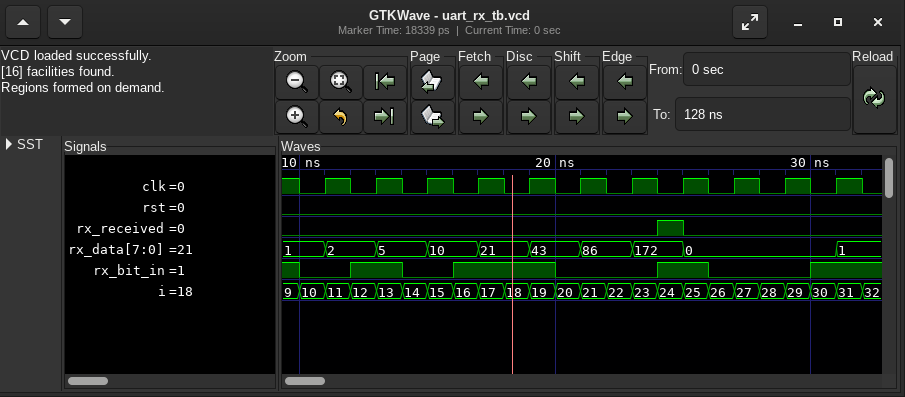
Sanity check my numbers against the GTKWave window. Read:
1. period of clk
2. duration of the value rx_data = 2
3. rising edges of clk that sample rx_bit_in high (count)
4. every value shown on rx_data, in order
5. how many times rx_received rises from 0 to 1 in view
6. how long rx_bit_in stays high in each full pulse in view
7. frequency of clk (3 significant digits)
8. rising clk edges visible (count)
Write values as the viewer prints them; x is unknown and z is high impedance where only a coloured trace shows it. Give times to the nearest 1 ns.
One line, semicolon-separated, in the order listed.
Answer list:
2 ns; 2 ns; 5; 1, 2, 5, 10, 21, 43, 86, 172, 0, 1; 1; 2 ns, 4 ns, 2 ns; 500 MHz; 11
